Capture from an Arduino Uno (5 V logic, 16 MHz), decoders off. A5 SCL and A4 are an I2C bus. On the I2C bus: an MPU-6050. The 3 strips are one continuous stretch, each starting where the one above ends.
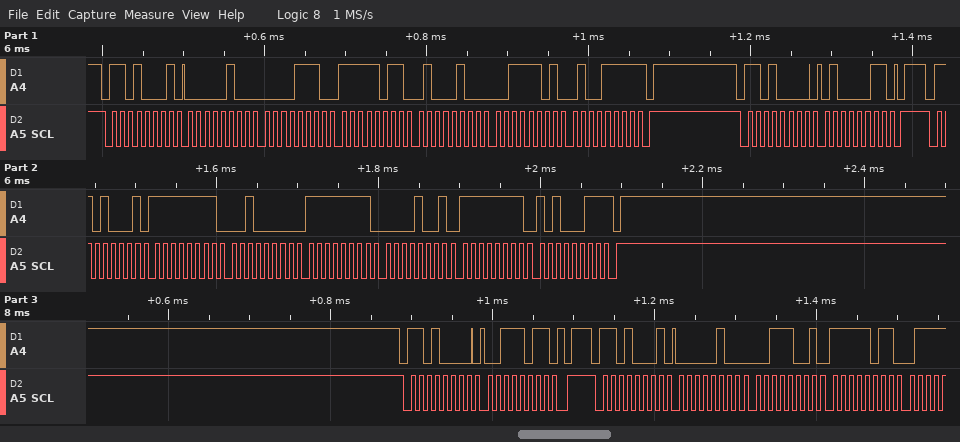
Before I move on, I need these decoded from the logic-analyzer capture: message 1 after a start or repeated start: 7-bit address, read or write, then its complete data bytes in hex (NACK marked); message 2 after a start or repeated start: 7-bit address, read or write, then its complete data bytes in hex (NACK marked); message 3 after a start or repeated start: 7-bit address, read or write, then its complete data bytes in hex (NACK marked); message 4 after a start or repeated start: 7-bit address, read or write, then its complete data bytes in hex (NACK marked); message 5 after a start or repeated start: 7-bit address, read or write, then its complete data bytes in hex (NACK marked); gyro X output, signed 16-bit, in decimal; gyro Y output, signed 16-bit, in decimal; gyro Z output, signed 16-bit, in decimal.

0x68 read: 04 0E FB 44 3D 4F NACK
0x68 write: 43
0x68 read: FF 20 FF 09 FF A3 NACK
0x68 write: 3B
0x68 read: 04 39 FB
-224
-247
-93
